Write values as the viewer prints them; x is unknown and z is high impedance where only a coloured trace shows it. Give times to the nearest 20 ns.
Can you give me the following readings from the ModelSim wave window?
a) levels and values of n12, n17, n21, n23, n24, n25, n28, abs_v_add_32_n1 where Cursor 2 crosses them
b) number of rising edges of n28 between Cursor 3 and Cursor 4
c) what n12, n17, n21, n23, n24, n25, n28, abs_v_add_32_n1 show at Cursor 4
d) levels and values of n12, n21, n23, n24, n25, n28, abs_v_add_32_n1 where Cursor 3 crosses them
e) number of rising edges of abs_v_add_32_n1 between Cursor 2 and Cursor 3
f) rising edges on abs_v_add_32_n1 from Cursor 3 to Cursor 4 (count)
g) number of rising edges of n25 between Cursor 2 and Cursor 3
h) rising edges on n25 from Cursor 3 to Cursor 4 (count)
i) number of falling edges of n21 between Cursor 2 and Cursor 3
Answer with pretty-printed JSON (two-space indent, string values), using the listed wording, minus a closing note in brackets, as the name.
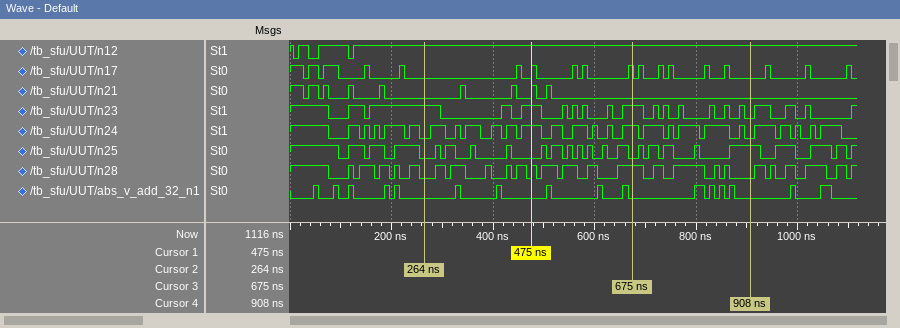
{
  "levels and values of n12, n17, n21, n23, n24, n25, n28, abs_v_add_32_n1 where Cursor 2 crosses them": "n12=1, n17=0, n21=0, n23=1, n24=0, n25=0, n28=0, abs_v_add_32_n1=0",
  "number of rising edges of n28 between Cursor 3 and Cursor 4": "4",
  "what n12, n17, n21, n23, n24, n25, n28, abs_v_add_32_n1 show at Cursor 4": "n12=1, n17=0, n21=0, n23=0, n24=0, n25=1, n28=0, abs_v_add_32_n1=0",
  "levels and values of n12, n21, n23, n24, n25, n28, abs_v_add_32_n1 where Cursor 3 crosses them": "n12=1, n21=0, n23=1, n24=1, n25=0, n28=1, abs_v_add_32_n1=0",
  "number of rising edges of abs_v_add_32_n1 between Cursor 2 and Cursor 3": "5",
  "rising edges on abs_v_add_32_n1 from Cursor 3 to Cursor 4": "4",
  "number of rising edges of n25 between Cursor 2 and Cursor 3": "11",
  "rising edges on n25 from Cursor 3 to Cursor 4": "5",
  "number of falling edges of n21 between Cursor 2 and Cursor 3": "4"
}
